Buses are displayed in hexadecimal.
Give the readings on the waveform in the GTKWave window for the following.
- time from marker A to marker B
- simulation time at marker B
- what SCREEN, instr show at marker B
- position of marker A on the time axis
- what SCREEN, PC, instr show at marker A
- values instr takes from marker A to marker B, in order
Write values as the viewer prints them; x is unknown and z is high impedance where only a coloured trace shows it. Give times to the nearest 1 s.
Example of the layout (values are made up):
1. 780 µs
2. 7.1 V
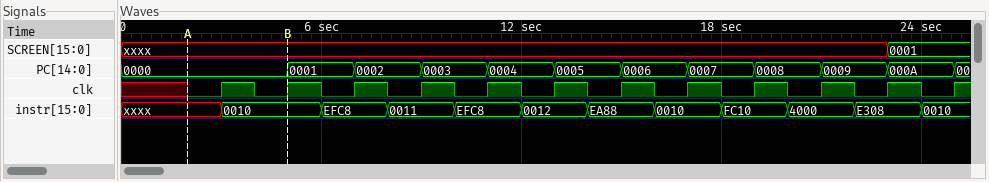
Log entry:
1. 3 s
2. 5 s
3. SCREEN=xxxx, instr=0010
4. 2 s
5. SCREEN=xxxx, PC=0000, instr=xxxx
6. xxxx, 0010
